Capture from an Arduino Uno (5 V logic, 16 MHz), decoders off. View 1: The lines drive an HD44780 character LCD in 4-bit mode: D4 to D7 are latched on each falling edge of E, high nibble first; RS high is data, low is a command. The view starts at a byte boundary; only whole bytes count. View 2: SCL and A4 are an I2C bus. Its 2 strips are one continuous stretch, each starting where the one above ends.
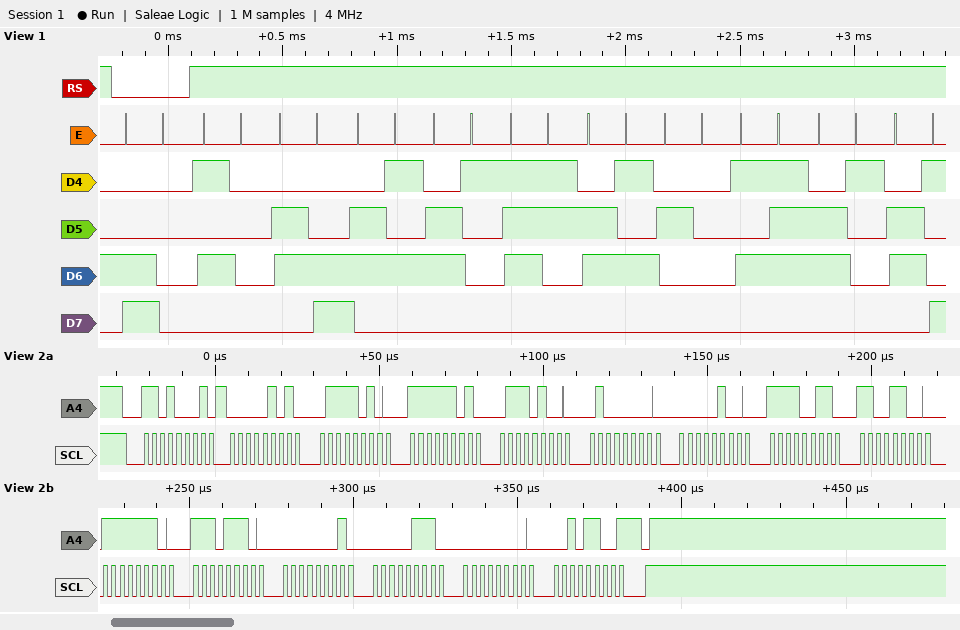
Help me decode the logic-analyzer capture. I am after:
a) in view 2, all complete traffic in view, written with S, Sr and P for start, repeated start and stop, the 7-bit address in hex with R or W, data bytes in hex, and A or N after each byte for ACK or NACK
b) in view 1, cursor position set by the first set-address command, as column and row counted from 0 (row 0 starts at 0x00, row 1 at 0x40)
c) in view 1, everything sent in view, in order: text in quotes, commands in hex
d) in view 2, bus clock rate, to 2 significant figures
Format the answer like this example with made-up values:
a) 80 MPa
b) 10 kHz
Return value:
a) S 68R A 05 A 7A A FD A 74 A 40 A 04 A F3 A CC A FE A EE A 01 A 07 A 00 A 2C N P
b) column 0, row 1
c) 0xC0 "Please Wai"
d) 400 kHz
